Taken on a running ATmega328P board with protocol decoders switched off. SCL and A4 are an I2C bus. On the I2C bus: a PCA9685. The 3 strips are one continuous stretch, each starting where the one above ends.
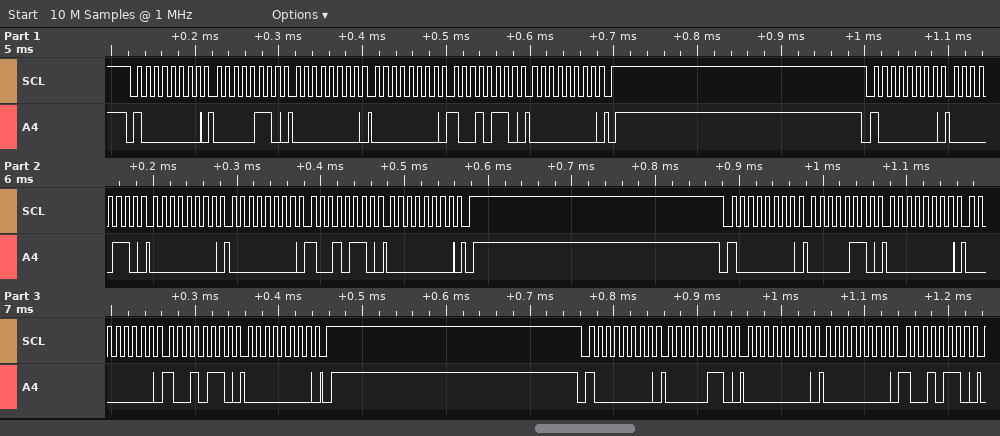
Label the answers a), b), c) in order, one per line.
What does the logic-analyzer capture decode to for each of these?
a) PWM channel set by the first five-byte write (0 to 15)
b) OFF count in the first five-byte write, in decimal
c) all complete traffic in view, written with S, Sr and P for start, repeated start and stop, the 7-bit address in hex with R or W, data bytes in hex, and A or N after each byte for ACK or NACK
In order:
a) 0
b) 150
c) S 40W A 06 A 00 A 00 A 96 A 00 A P S 40W A 06 A 00 A 00 A 96 A 00 A P S 40W A 06 A 00 A 00 A 96 A 00 A P S 40W A 06 A 00 A 00 A 96 A
